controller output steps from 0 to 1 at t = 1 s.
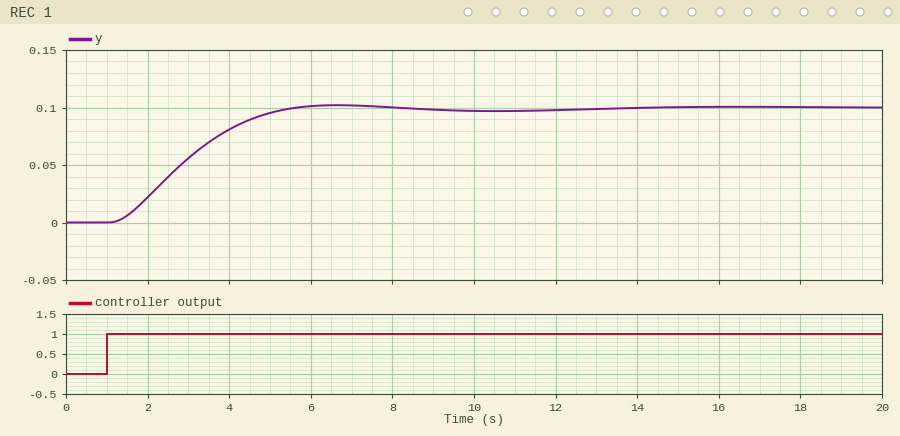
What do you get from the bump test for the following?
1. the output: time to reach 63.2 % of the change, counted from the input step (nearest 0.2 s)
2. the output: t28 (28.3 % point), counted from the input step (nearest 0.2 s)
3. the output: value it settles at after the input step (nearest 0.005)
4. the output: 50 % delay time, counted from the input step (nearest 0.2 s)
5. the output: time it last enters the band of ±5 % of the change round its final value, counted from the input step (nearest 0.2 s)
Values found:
2.2 s
1.2 s
0.100
1.8 s
4.0 s
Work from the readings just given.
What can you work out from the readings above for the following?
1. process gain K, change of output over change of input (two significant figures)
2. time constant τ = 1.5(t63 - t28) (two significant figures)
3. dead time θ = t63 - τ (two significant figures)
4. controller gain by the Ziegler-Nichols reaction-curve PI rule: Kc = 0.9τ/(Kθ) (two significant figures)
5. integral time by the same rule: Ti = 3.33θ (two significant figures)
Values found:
0.10
1.5 s
0.70 s
19
2.3 s
